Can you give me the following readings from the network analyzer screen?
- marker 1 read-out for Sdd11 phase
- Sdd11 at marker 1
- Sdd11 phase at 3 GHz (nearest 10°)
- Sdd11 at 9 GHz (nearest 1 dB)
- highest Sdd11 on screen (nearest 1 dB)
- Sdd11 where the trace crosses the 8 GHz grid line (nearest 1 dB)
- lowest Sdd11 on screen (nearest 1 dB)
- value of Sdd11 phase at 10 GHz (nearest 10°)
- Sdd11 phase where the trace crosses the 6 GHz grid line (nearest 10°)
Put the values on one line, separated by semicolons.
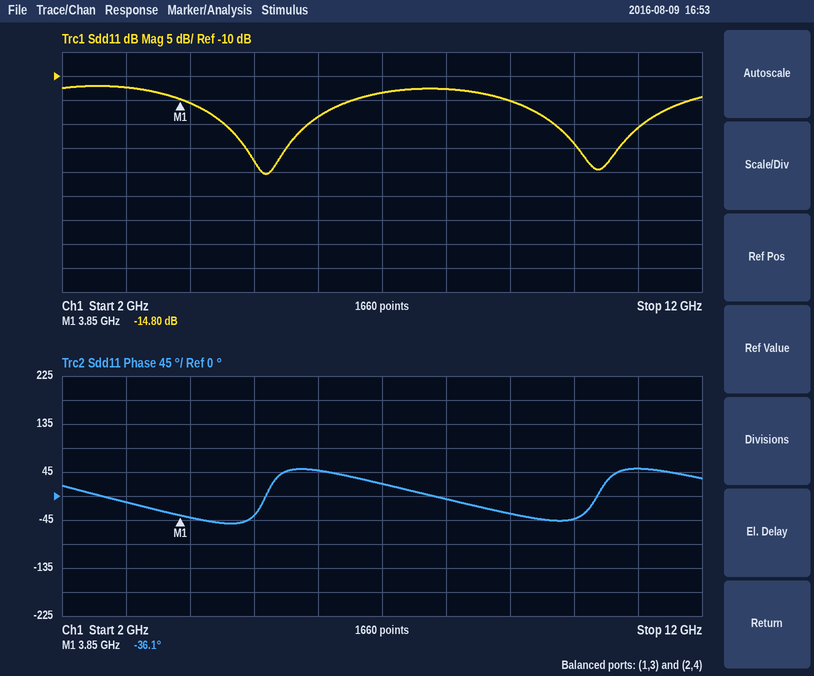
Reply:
-36.1°; -14.80 dB; -10°; -15 dB; -12 dB; -13 dB; -30 dB; -40°; 50°
